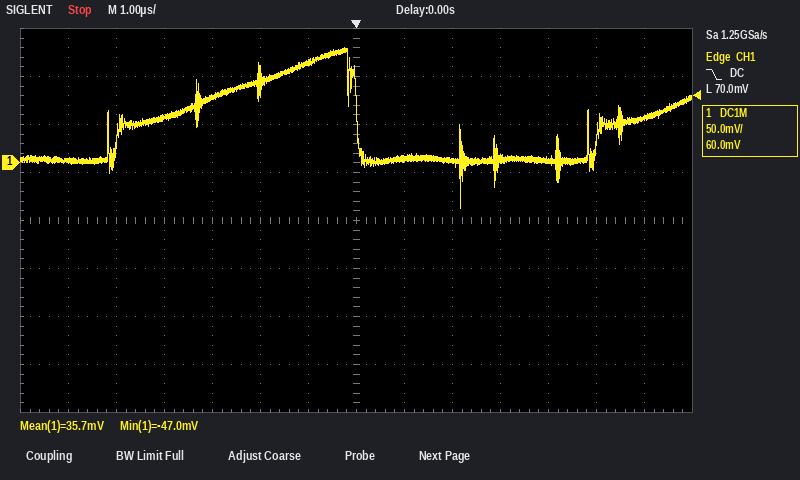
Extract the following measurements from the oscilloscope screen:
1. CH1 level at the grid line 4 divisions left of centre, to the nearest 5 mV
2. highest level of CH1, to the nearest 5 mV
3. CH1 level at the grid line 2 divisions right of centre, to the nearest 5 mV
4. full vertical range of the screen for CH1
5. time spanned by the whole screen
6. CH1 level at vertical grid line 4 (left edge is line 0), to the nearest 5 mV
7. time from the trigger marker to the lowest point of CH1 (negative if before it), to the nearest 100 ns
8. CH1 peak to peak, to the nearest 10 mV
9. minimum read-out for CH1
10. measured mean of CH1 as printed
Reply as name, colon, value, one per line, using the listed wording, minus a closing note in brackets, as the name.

CH1 level at the grid line 4 divisions left of centre, to the nearest 5 mV: 45 mV
highest level of CH1, to the nearest 5 mV: 120 mV
CH1 level at the grid line 2 divisions right of centre, to the nearest 5 mV: 0 mV
full vertical range of the screen for CH1: 400 mV
time spanned by the whole screen: 14 µs
CH1 level at vertical grid line 4 (left edge is line 0), to the nearest 5 mV: 70 mV
time from the trigger marker to the lowest point of CH1 (negative if before it), to the nearest 100 ns: +2.2 µs
CH1 peak to peak, to the nearest 10 mV: 170 mV
minimum read-out for CH1: -47.0 mV
measured mean of CH1 as printed: 35.7 mV
